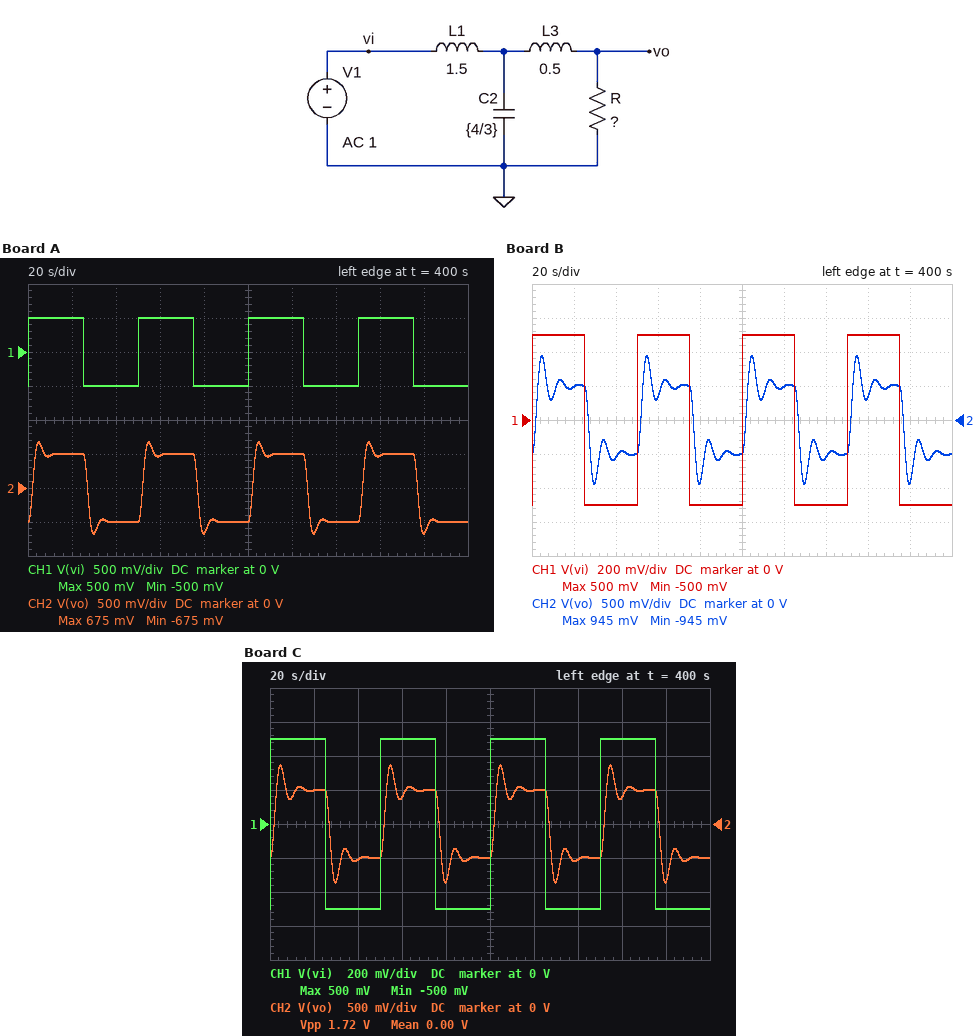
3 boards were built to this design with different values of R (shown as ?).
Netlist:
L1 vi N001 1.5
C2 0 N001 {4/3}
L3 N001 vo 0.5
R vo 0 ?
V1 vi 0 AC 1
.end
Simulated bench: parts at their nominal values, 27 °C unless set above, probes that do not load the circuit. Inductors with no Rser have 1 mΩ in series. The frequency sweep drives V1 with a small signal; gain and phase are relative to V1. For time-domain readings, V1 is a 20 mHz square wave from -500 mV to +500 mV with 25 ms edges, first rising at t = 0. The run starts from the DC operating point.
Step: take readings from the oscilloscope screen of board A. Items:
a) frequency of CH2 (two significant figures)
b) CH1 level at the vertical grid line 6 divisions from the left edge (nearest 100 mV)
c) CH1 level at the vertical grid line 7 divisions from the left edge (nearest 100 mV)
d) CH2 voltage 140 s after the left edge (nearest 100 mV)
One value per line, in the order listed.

20 mHz
500 mV
-500 mV
-500 mV
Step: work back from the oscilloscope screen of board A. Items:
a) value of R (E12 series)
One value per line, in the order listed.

1.2 Ω
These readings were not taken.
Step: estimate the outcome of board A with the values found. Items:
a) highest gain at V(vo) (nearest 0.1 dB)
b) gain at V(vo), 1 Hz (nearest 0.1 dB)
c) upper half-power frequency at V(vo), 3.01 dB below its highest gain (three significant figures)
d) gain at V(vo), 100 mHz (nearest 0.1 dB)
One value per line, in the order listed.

1.2 dB
-46.5 dB
154 mHz
1.2 dB
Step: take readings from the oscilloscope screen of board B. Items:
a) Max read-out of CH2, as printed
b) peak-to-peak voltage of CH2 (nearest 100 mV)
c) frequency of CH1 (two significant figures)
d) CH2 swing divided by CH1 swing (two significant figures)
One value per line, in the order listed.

945 mV
1.9 V
20 mHz
1.9
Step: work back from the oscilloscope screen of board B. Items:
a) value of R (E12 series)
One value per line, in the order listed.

2.2 Ω
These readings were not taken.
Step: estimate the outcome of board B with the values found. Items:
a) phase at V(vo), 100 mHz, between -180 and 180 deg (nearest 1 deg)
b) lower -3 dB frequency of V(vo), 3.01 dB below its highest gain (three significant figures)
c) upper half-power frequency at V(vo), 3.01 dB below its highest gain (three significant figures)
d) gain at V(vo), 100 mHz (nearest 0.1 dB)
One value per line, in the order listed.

-65 deg
74.2 mHz
136 mHz
5.9 dB
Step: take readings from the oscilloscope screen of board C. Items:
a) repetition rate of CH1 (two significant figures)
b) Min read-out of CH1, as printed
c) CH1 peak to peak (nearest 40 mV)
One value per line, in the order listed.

20 mHz
-500 mV
1.00 V
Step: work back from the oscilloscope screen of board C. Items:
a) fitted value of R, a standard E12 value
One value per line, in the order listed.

1.8 Ω
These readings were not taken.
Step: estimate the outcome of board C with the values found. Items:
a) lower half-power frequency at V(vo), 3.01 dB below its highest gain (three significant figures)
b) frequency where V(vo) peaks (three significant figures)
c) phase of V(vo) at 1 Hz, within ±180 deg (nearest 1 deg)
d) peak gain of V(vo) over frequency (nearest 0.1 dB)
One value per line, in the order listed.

57.5 mHz
108 mHz
121 deg
4.6 dB
